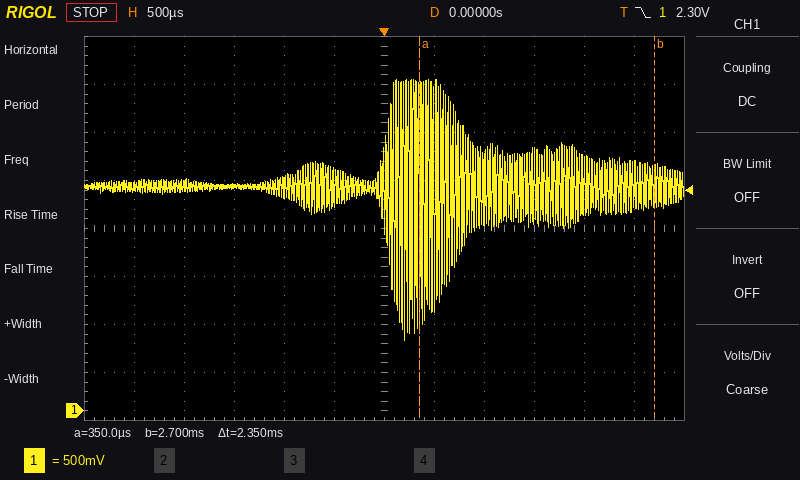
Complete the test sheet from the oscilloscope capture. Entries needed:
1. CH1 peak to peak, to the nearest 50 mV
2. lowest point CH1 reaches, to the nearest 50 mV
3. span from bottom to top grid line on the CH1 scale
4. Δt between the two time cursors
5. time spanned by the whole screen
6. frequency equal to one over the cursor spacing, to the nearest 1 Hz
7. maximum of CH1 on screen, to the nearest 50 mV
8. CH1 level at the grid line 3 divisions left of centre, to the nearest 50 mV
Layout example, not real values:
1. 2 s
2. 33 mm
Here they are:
1. 2.70 V
2. 750 mV
3. 4 V
4. 2.35 ms
5. 6 ms
6. 426 Hz
7. 3.45 V
8. 2.35 V
